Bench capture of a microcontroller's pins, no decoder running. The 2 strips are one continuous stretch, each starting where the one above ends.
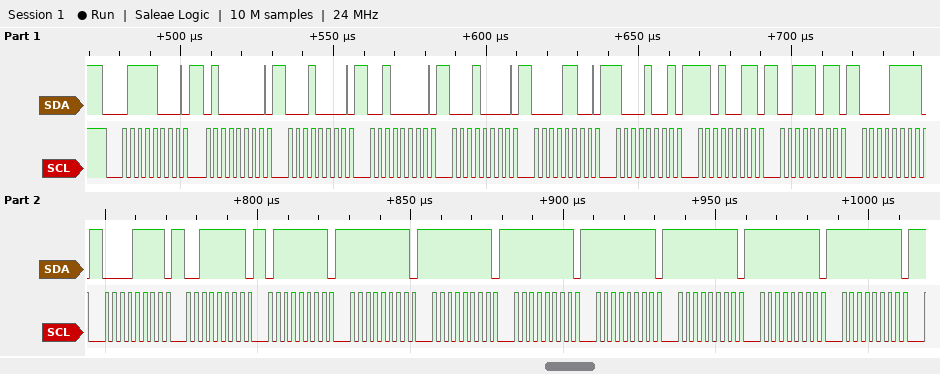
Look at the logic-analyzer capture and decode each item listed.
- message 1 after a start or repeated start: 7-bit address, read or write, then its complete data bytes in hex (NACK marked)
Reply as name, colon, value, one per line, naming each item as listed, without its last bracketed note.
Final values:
message 1 after a start or repeated start: 7-bit address, read or write, then its complete data bytes in hex: 0x3C write: 40 10 20 10 0C 89 D3 3B 0F 0F 3F 7F FF FF FF FF FF FF FF
